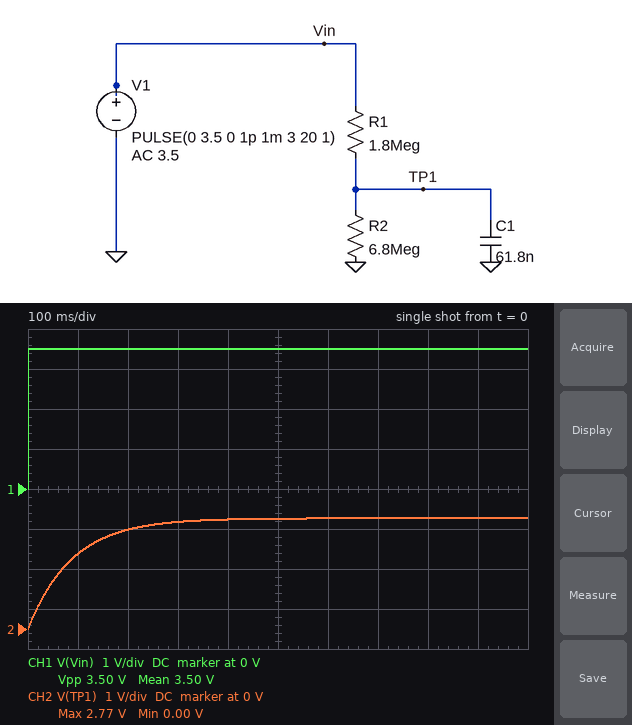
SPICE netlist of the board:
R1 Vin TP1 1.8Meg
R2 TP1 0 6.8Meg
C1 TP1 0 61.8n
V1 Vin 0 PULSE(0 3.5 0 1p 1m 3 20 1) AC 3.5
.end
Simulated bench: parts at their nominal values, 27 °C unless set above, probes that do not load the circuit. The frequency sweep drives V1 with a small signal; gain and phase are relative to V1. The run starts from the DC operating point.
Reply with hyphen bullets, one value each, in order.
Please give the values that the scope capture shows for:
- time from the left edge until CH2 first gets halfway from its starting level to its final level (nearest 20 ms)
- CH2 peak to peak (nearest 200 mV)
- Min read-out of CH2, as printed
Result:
- 60 ms
- 2.8 V
- 0.00 V
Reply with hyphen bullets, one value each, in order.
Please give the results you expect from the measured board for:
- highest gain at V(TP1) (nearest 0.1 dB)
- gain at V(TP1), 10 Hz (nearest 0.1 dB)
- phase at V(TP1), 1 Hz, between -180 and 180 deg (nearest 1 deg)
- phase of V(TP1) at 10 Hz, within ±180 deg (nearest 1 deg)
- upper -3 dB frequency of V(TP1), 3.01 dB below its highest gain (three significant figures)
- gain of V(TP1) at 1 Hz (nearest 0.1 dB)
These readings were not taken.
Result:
- -2.0 dB
- -17.0 dB
- -29 deg
- -80 deg
- 1.81 Hz
- -3.2 dB
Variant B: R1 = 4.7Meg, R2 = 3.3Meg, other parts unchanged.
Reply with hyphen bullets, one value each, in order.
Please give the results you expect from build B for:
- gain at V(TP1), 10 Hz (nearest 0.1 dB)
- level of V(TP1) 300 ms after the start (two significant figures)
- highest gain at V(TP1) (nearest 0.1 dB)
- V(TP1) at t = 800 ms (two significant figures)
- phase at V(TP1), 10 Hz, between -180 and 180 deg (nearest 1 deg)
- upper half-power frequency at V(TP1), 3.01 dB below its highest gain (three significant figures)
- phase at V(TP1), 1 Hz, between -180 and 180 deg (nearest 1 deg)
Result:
- -25.3 dB
- 1.3 V
- -7.7 dB
- 1.4 V
- -82 deg
- 1.33 Hz
- -37 deg
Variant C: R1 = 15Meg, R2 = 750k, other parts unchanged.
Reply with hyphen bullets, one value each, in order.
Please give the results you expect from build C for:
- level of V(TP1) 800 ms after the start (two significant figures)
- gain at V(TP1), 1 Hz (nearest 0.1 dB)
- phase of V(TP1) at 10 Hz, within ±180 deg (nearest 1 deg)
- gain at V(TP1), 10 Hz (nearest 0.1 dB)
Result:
- 170 mV
- -26.8 dB
- -70 deg
- -35.8 dB
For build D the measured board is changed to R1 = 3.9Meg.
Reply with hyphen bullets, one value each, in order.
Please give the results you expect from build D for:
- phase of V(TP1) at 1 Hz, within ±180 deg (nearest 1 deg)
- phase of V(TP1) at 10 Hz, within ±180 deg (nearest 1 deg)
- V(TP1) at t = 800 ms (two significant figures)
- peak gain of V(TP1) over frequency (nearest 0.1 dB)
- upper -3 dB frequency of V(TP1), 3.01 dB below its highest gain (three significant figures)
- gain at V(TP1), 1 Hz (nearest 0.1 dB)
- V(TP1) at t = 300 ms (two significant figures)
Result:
- -44 deg
- -84 deg
- 2.2 V
- -3.9 dB
- 1.04 Hz
- -6.8 dB
- 1.9 V
